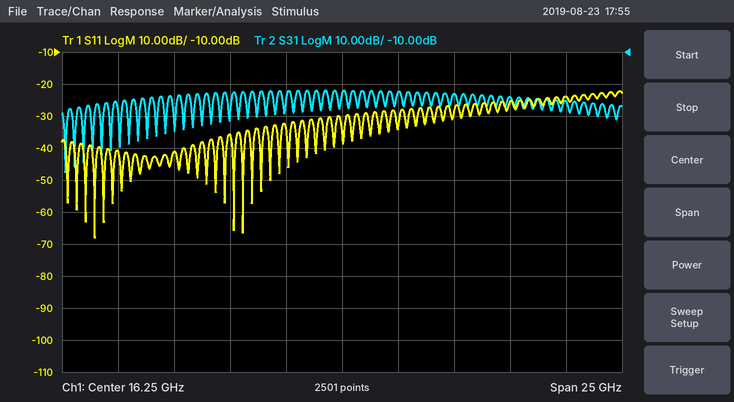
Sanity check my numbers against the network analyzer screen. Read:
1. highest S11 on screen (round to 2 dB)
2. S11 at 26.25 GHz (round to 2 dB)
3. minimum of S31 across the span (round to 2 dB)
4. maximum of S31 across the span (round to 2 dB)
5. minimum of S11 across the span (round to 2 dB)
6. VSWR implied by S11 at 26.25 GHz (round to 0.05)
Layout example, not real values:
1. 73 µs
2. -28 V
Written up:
1. -22 dB
2. -24 dB
3. -48 dB
4. -22 dB
5. -68 dB
6. 1.15
